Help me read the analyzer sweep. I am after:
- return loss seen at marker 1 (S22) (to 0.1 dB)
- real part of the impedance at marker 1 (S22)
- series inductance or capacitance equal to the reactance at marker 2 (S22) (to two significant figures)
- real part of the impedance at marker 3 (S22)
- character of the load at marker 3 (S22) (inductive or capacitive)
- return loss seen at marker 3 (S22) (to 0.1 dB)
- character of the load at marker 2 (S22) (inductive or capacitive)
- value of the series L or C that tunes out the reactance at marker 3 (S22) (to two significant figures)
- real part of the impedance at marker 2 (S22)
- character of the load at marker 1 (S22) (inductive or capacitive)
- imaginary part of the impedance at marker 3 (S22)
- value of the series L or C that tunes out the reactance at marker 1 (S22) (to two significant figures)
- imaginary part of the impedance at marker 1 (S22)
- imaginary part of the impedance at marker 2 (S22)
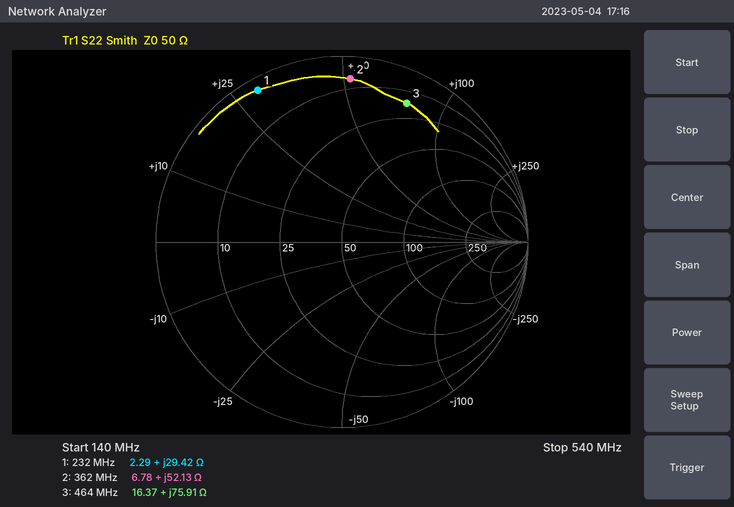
0.6 dB
2.29 Ω
23 nH
16.37 Ω
inductive
1.7 dB
inductive
4.5 pF
6.78 Ω
inductive
+75.91 Ω
23 pF
+29.42 Ω
+52.13 Ω
